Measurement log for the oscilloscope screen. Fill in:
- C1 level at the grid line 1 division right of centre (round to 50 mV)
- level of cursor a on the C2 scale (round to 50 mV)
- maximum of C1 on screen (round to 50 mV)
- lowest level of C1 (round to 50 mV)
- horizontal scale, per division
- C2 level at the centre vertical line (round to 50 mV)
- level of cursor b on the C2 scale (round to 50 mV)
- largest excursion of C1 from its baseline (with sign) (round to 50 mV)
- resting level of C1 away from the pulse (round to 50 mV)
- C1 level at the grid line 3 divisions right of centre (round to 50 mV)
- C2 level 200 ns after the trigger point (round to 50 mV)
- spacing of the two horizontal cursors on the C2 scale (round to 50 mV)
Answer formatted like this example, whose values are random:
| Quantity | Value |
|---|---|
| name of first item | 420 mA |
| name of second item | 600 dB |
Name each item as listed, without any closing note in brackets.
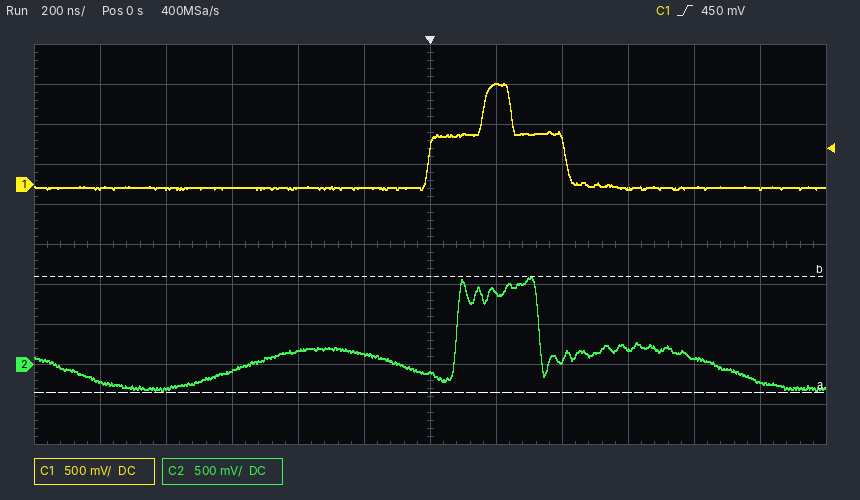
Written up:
| Quantity | Value |
|---|---|
| C1 level at the grid line 1 division right of centre | 1.25 V |
| level of cursor a on the C2 scale | -350 mV |
| maximum of C1 on screen | 1.25 V |
| lowest level of C1 | -50 mV |
| horizontal scale, per division | 200 ns |
| C2 level at the centre vertical line | -100 mV |
| level of cursor b on the C2 scale | 1.10 V |
| largest excursion of C1 from its baseline (with sign) | +1.30 V |
| resting level of C1 away from the pulse | -50 mV |
| C1 level at the grid line 3 divisions right of centre | -50 mV |
| C2 level 200 ns after the trigger point | 900 mV |
| spacing of the two horizontal cursors on the C2 scale | 1.45 V |
